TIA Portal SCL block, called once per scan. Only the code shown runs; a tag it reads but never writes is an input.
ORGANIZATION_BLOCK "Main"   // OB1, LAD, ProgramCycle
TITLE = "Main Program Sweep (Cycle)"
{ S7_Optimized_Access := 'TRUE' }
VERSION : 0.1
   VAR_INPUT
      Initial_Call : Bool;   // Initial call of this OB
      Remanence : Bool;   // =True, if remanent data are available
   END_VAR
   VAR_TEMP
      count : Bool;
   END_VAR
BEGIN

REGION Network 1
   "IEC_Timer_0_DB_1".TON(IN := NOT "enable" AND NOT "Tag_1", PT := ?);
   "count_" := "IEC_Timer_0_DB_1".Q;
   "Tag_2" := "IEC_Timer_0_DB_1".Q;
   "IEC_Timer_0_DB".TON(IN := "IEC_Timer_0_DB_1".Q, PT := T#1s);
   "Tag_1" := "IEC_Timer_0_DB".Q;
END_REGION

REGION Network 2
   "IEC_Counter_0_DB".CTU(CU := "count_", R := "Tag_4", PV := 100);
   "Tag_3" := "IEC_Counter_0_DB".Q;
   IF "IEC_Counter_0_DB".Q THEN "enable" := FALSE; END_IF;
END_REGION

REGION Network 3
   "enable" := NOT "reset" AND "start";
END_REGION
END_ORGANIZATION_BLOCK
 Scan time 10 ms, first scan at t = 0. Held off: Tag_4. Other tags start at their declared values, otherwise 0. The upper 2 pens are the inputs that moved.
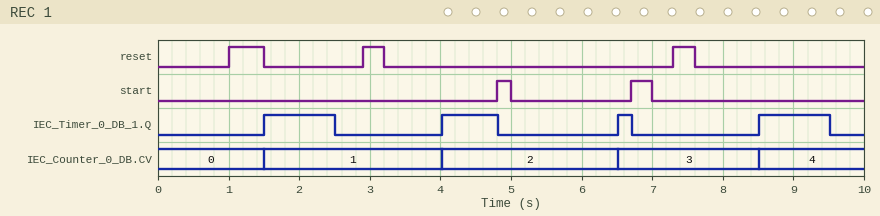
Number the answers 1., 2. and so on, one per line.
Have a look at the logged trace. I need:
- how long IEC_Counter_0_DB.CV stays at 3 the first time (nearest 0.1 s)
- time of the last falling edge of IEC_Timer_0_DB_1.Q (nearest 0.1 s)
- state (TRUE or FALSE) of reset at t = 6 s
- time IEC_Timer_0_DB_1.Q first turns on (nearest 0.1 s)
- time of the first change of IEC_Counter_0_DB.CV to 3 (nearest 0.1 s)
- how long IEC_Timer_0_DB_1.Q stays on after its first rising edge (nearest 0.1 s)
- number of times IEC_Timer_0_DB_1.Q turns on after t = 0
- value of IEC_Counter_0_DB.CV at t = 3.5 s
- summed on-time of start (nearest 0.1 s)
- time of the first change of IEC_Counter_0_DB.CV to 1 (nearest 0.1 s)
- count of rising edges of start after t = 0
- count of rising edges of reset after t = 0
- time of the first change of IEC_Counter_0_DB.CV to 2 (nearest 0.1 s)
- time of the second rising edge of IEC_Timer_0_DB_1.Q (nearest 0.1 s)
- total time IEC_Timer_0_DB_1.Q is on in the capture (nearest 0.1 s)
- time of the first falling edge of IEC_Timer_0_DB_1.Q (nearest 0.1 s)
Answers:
1. 2.0 s
2. 9.5 s
3. FALSE
4. 1.5 s
5. 6.5 s
6. 1.0 s
7. 4
8. 1
9. 0.5 s
10. 1.5 s
11. 2
12. 3
13. 4.0 s
14. 4.0 s
15. 3.0 s
16. 2.5 s
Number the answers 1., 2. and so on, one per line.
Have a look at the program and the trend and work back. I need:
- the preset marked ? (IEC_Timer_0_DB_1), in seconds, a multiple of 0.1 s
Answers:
1. 1.5 s
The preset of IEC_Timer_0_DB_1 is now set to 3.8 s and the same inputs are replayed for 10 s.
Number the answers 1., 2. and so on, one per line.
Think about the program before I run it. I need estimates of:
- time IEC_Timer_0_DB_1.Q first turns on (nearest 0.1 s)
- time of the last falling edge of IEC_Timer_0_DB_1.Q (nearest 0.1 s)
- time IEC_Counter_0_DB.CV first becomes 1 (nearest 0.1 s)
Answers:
1. 3.8 s
2. 4.8 s
3. 3.8 s
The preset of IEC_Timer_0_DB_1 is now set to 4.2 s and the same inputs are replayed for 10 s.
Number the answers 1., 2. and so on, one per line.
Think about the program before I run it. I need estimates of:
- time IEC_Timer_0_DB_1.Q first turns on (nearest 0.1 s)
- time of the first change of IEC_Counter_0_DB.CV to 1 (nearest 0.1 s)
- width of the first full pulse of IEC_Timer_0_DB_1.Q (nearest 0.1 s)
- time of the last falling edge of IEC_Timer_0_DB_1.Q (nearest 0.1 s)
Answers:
1. 4.2 s
2. 4.2 s
3. 0.6 s
4. 4.8 s
